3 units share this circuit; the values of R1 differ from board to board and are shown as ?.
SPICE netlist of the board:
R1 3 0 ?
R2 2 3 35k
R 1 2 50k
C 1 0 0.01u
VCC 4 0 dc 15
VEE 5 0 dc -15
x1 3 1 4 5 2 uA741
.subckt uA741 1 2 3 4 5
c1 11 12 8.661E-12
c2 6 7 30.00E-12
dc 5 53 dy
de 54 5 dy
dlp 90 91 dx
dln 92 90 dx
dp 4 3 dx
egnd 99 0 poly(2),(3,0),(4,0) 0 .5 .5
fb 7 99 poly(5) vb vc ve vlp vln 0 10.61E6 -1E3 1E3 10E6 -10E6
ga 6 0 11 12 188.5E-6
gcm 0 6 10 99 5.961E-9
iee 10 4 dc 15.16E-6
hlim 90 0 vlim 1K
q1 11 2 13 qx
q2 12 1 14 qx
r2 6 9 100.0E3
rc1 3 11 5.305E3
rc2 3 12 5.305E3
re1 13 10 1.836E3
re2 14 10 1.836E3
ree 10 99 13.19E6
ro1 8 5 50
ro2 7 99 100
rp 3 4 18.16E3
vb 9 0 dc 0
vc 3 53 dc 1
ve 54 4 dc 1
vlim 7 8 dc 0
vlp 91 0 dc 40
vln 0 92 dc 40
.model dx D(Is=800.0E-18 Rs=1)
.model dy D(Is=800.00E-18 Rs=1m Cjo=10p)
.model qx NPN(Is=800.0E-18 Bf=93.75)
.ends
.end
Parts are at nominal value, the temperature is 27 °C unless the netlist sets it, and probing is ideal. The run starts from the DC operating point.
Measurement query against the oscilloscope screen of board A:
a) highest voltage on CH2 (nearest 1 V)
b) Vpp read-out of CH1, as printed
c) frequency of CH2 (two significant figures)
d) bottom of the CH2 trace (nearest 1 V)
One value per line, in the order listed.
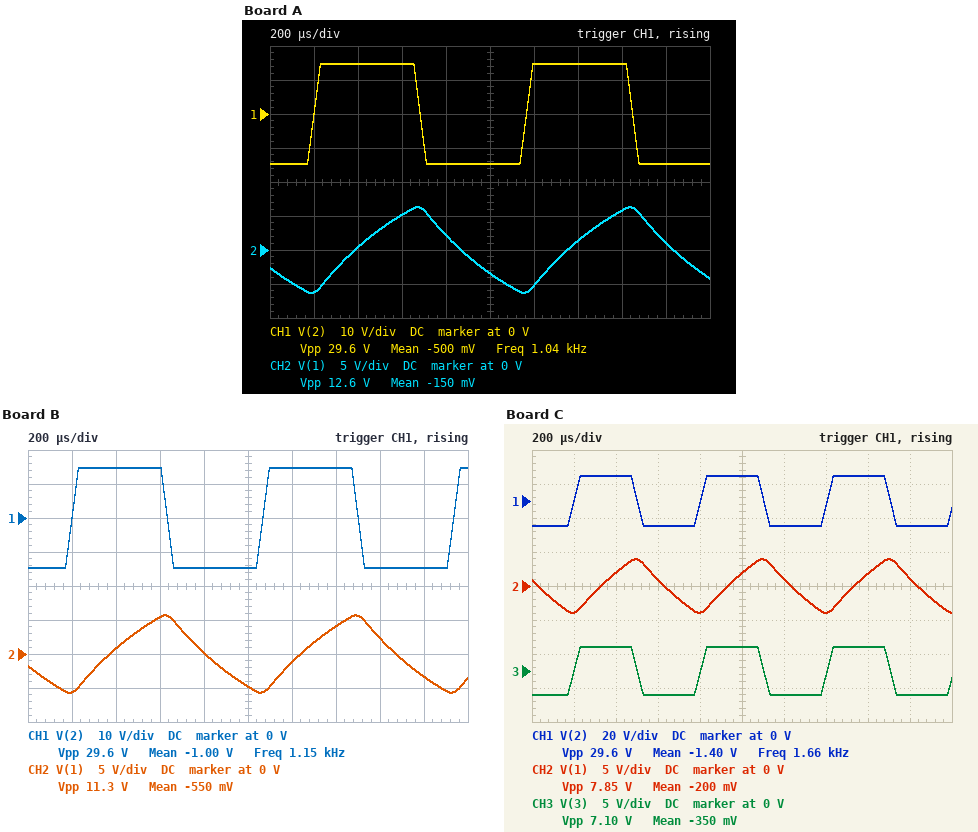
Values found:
6 V
29.6 V
1.0 kHz
-6 V
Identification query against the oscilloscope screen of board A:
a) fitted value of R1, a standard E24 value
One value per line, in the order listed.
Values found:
24 kΩ
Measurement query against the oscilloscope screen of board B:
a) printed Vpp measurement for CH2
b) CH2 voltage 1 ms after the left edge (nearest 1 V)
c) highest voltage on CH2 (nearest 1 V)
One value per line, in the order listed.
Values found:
11.3 V
-5 V
6 V
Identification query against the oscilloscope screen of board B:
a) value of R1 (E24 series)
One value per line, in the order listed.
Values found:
20 kΩ
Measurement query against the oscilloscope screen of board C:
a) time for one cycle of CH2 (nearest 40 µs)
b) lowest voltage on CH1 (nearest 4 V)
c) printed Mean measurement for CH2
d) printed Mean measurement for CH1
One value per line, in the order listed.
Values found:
600 µs
-16 V
-200 mV
-1.40 V
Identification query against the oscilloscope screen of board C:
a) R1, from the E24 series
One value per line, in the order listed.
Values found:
11 kΩ
